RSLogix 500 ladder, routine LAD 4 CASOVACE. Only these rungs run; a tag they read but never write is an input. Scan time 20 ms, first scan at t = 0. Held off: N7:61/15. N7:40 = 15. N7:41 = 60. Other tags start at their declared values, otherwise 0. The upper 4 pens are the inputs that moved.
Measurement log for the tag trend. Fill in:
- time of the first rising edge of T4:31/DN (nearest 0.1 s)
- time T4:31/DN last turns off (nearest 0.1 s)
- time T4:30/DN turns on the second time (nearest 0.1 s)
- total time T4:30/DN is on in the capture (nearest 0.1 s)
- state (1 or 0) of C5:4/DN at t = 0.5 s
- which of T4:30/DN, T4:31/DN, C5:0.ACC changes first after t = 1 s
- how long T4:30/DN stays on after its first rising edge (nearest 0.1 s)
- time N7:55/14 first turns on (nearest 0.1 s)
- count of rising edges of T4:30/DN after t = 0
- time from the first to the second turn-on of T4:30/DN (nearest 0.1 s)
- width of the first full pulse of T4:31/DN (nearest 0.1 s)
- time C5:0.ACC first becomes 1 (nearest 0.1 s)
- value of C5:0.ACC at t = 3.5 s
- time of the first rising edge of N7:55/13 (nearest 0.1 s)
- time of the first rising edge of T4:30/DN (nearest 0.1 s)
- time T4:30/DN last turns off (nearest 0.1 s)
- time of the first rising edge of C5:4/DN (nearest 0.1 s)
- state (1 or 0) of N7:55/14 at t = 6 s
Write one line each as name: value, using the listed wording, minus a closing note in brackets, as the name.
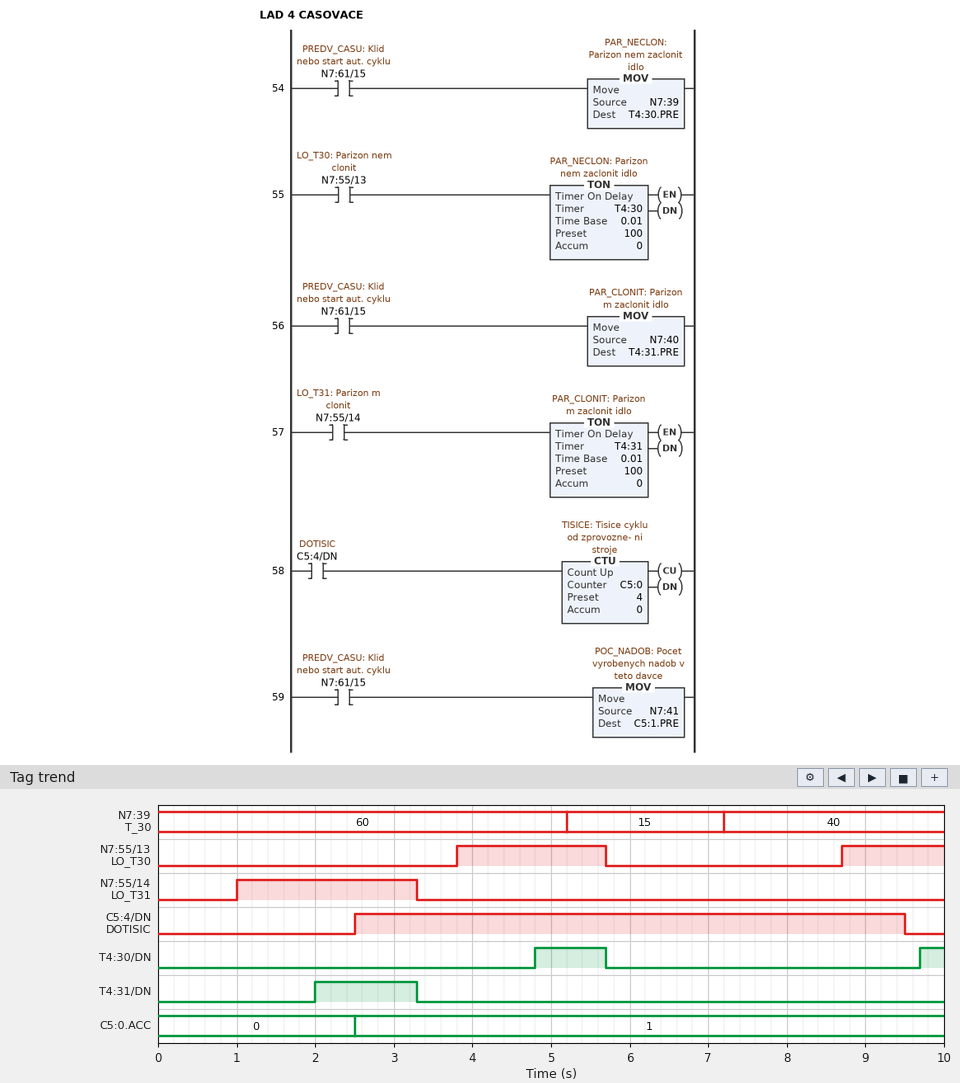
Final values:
time of the first rising edge of T4:31/DN: 2.0 s
time T4:31/DN last turns off: 3.3 s
time T4:30/DN turns on the second time: 9.7 s
total time T4:30/DN is on in the capture: 1.2 s
state (1 or 0) of C5:4/DN at t = 0.5 s: 0
which of T4:30/DN, T4:31/DN, C5:0.ACC changes first after t = 1 s: T4:31/DN
how long T4:30/DN stays on after its first rising edge: 0.9 s
time N7:55/14 first turns on: 1.0 s
count of rising edges of T4:30/DN after t = 0: 2
time from the first to the second turn-on of T4:30/DN: 4.9 s
width of the first full pulse of T4:31/DN: 1.3 s
time C5:0.ACC first becomes 1: 2.5 s
value of C5:0.ACC at t = 3.5 s: 1
time of the first rising edge of N7:55/13: 3.8 s
time of the first rising edge of T4:30/DN: 4.8 s
time T4:30/DN last turns off: 5.7 s
time of the first rising edge of C5:4/DN: 2.5 s
state (1 or 0) of N7:55/14 at t = 6 s: 0
